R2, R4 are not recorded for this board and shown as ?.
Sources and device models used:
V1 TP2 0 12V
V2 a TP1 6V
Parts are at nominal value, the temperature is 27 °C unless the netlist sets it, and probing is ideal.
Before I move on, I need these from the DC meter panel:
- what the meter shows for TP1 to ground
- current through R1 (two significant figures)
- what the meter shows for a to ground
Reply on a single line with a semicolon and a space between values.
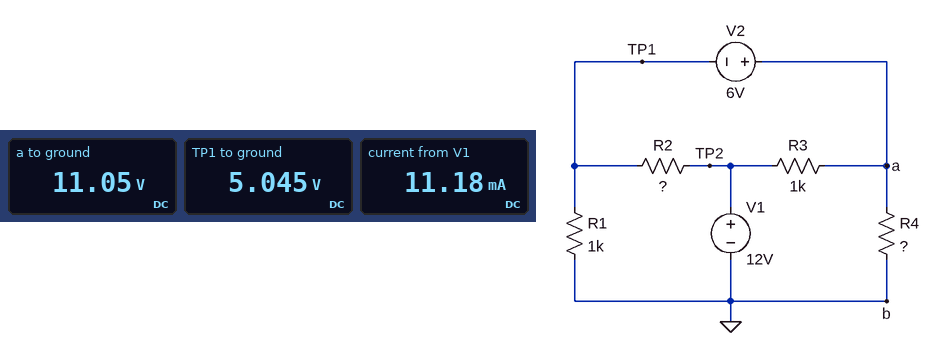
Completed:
5.045 V; 5.0 mA; 11.05 V
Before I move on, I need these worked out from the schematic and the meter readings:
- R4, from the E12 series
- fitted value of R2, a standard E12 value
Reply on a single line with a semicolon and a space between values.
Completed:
1.8 kΩ; 680 Ω
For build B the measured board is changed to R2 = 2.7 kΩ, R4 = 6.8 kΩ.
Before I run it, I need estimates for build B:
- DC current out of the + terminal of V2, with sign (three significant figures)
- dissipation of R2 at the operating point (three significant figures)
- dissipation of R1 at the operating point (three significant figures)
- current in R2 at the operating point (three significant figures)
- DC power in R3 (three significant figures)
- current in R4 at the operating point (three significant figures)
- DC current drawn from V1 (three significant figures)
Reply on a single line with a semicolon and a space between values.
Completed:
-761 µA; 24.9 mW; 14.4 mW; 3.04 mA; 4.85 mW; 1.44 mA; 5.24 mA
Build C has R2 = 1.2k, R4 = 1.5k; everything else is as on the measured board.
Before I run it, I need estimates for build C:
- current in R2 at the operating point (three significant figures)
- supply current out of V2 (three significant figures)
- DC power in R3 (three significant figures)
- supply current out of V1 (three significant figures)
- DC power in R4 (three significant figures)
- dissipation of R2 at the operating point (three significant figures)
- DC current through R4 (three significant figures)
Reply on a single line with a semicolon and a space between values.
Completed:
7.14 mA; 3.71 mA; 6.61 mW; 9.71 mA; 59.3 mW; 61.2 mW; 6.29 mA
